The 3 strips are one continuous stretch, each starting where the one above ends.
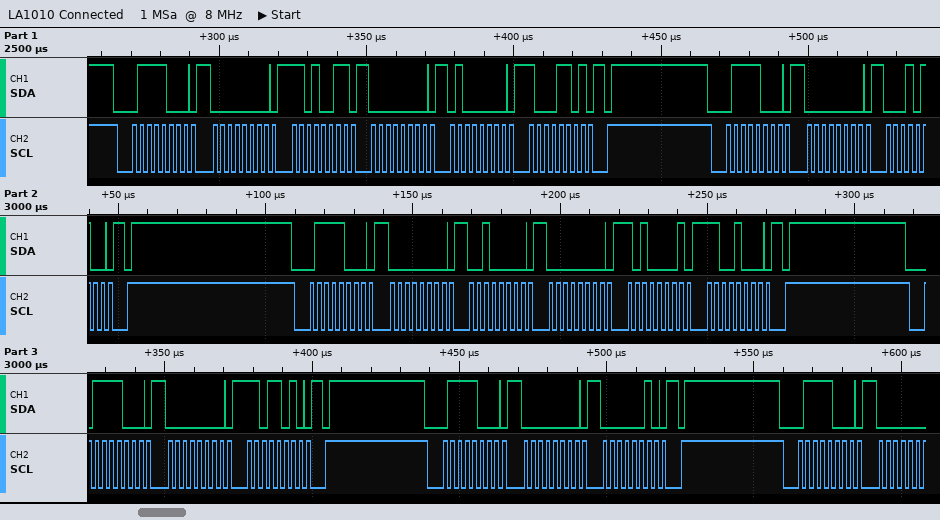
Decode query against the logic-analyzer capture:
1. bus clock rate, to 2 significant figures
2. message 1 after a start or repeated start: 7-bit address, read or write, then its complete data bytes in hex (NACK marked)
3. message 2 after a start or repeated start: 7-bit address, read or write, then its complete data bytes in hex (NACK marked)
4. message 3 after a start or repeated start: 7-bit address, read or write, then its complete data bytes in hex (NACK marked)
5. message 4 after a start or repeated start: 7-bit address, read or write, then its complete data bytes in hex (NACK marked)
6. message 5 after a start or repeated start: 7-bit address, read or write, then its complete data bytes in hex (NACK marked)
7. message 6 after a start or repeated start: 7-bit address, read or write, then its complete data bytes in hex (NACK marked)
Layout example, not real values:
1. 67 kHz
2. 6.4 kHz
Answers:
1. 400 kHz
2. 0x3C write: 00 D3 00 40 8D
3. 0x3C write: 00 14
4. 0x3C write: 00 20 00 A1 C8
5. 0x3C write: 00 DA
6. 0x3C write: 00 02
7. 0x3C write
